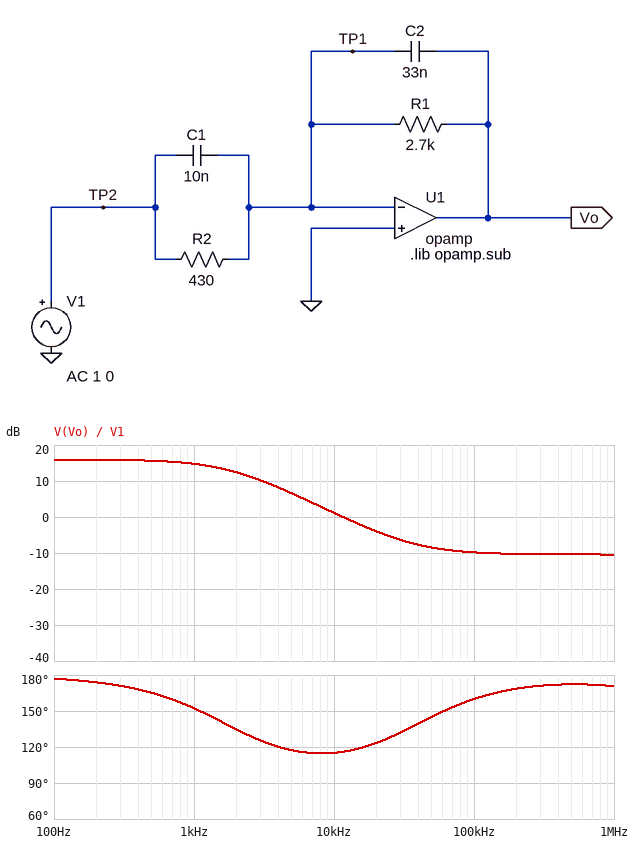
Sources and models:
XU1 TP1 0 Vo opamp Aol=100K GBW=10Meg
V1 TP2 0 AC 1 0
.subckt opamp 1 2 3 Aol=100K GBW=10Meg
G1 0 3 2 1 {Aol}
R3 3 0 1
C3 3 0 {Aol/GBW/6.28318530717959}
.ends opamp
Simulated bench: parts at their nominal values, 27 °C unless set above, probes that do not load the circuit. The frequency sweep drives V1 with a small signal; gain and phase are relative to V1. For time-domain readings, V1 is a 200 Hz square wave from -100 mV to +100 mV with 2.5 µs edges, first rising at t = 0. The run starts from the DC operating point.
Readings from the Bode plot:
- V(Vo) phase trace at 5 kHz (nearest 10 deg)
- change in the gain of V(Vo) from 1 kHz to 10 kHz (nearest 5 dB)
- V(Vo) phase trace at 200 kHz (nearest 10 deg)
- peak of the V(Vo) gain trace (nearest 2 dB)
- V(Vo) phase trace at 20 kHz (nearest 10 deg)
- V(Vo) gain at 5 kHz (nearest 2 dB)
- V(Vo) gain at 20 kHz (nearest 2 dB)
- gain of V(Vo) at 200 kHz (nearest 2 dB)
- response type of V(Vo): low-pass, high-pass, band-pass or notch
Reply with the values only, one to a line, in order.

120 deg
-15 dB
170 deg
16 dB
120 deg
6 dB
-4 dB
-10 dB
low-pass
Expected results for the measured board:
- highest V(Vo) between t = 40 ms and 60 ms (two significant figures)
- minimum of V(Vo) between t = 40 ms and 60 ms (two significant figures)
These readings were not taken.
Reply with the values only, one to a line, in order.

630 mV
-630 mV
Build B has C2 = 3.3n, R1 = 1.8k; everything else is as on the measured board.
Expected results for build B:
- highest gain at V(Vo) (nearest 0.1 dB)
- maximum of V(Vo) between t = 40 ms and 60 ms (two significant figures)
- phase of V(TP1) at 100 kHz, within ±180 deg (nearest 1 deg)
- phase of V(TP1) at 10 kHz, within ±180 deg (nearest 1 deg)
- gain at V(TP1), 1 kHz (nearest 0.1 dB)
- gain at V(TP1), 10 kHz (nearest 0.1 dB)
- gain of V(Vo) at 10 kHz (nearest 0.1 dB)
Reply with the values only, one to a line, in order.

12.4 dB
420 mV
82 deg
84 deg
-67.5 dB
-47.8 dB
12.2 dB
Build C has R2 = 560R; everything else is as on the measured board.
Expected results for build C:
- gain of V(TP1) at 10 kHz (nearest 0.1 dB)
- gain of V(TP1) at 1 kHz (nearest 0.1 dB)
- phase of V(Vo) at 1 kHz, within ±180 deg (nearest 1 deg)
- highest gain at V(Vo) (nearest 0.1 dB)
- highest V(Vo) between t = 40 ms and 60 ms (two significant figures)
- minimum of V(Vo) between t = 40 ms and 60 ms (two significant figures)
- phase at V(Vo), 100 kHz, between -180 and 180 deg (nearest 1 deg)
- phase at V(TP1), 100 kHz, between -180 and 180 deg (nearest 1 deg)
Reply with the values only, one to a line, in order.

-60.9 dB
-67.5 dB
153 deg
13.7 dB
480 mV
-480 mV
164 deg
74 deg
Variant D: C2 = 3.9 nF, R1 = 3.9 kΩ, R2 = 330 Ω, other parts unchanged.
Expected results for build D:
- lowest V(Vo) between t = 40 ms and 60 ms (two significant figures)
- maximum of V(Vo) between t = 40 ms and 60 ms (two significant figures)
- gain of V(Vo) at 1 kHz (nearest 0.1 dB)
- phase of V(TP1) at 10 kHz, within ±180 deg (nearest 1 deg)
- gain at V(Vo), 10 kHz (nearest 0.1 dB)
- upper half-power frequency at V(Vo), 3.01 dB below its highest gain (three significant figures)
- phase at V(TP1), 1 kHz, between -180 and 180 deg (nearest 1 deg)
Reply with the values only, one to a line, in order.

-1.2 V
1.2 V
21.4 dB
57 deg
18.8 dB
10.9 kHz
80 deg
